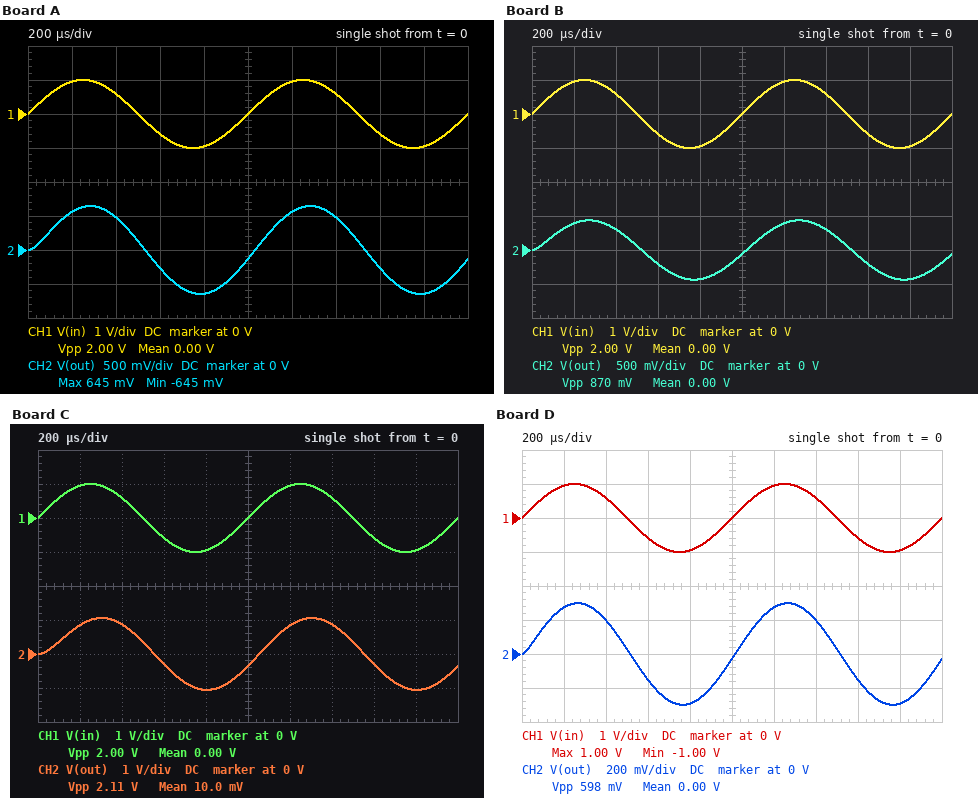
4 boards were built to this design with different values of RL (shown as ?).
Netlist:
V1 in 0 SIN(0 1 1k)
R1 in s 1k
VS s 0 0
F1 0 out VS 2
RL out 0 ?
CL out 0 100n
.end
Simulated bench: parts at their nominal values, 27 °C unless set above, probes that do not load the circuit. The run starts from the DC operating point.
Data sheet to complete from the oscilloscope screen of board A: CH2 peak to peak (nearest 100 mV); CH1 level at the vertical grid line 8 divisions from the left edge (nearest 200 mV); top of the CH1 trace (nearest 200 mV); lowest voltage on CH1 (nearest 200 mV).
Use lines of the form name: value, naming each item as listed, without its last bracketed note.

CH2 peak to peak: 1.3 V
CH1 level at the vertical grid line 8 divisions from the left edge: -600 mV
top of the CH1 trace: 1.0 V
lowest voltage on CH1: -1.0 V
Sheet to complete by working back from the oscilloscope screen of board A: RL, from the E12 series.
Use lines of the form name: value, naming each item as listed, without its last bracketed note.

RL, from the E12 series: 330 Ω
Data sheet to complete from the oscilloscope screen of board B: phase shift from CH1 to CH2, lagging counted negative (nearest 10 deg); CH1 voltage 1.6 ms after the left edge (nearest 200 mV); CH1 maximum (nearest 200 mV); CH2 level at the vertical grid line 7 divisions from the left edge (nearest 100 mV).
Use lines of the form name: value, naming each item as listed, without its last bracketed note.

phase shift from CH1 to CH2, lagging counted negative: -10 deg
CH1 voltage 1.6 ms after the left edge: -600 mV
CH1 maximum: 1.0 V
CH2 level at the vertical grid line 7 divisions from the left edge: 300 mV
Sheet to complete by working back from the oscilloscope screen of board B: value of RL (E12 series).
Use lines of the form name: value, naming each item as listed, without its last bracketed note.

value of RL: 220 Ω
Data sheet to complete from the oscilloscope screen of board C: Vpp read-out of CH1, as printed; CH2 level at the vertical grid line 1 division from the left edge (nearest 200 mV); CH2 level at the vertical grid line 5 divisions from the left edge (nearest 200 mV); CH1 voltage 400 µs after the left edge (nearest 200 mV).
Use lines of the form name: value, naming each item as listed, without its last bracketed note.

Vpp read-out of CH1, as printed: 2.00 V
CH2 level at the vertical grid line 1 division from the left edge: 800 mV
CH2 level at the vertical grid line 5 divisions from the left edge: -400 mV
CH1 voltage 400 µs after the left edge: 600 mV
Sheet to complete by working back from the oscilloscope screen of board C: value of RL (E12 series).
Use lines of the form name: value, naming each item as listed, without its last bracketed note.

value of RL: 560 Ω
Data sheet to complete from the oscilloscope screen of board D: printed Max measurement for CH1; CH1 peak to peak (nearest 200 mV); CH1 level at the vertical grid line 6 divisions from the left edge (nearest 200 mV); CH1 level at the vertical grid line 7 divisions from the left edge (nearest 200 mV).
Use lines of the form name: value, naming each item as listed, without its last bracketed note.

printed Max measurement for CH1: 1.00 V
CH1 peak to peak: 2.0 V
CH1 level at the vertical grid line 6 divisions from the left edge: 1.0 V
CH1 level at the vertical grid line 7 divisions from the left edge: 600 mV
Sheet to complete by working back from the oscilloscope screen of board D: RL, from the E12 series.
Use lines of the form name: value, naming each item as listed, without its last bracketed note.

RL, from the E12 series: 150 Ω
